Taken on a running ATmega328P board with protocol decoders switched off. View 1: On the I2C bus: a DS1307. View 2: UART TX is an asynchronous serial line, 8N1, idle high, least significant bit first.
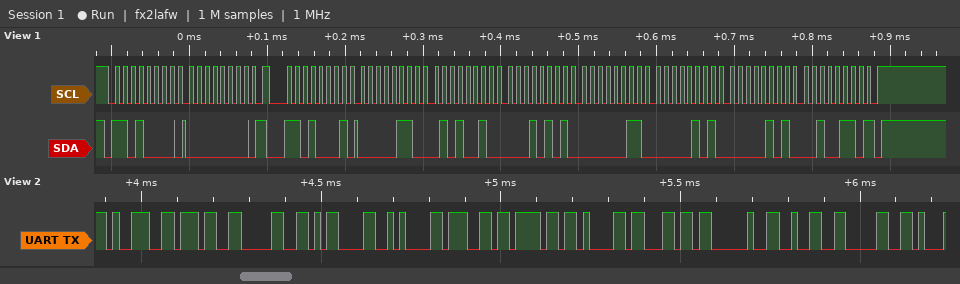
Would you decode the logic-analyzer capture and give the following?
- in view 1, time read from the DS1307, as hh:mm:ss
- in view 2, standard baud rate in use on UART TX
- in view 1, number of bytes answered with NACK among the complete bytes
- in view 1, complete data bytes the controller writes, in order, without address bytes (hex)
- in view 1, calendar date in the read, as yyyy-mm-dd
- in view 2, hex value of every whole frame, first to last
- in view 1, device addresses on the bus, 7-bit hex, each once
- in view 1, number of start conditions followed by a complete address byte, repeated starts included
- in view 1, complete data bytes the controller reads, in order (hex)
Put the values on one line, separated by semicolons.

15:52:06; 57600 baud; 1; 00; 2026-05-05; 0x39 0x37 0x30 0x0D 0x0A 0x67 0x6F 0x61 0x6C 0x20 0x32 0x30; 0x68; 2; 06 52 15 03 05 05 26
